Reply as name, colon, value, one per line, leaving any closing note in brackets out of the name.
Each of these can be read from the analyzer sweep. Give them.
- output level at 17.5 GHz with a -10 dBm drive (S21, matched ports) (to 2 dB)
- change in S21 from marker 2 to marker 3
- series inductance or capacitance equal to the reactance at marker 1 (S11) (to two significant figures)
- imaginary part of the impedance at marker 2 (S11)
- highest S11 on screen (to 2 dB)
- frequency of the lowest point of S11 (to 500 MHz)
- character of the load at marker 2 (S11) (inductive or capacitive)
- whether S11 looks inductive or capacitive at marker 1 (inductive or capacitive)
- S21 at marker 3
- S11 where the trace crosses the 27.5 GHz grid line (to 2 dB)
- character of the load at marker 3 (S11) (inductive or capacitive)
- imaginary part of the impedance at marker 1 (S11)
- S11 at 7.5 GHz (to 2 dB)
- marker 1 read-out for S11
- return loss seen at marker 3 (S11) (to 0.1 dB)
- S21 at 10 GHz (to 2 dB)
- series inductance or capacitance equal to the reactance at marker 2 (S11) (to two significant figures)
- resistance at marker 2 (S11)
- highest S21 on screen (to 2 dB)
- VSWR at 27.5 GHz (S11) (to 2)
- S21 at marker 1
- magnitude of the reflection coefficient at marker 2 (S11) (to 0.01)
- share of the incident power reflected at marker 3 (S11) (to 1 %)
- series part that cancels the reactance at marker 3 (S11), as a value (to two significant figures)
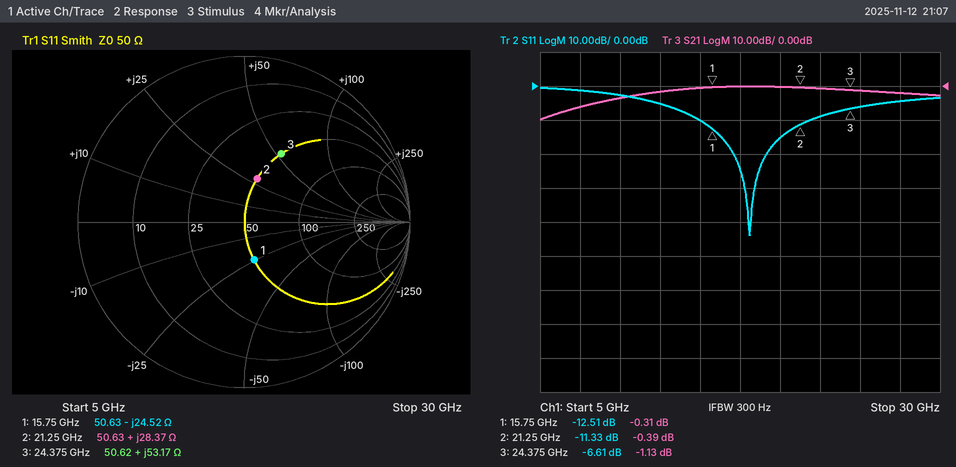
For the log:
output level at 17.5 GHz with a -10 dBm drive (S21, matched ports): -10 dBm
change in S21 from marker 2 to marker 3: -0.74 dB
series inductance or capacitance equal to the reactance at marker 1 (S11): 410 fF
imaginary part of the impedance at marker 2: +28.37 Ω
highest S11 on screen: 0 dB
frequency of the lowest point of S11: 18.0 GHz
character of the load at marker 2 (S11): inductive
whether S11 looks inductive or capacitive at marker 1: capacitive
S21 at marker 3: -1.13 dB
S11 where the trace crosses the 27.5 GHz grid line: -4 dB
character of the load at marker 3 (S11): inductive
imaginary part of the impedance at marker 1: -24.52 Ω
S11 at 7.5 GHz: -2 dB
marker 1 read-out for S11: -12.51 dB
return loss seen at marker 3 (S11): 6.6 dB
S21 at 10 GHz: -4 dB
series inductance or capacitance equal to the reactance at marker 2 (S11): 210 pH
resistance at marker 2: 50.63 Ω
highest S21 on screen: 0 dB
VSWR at 27.5 GHz (S11): 4
S21 at marker 1: -0.31 dB
magnitude of the reflection coefficient at marker 2 (S11): 0.27
share of the incident power reflected at marker 3 (S11): 22 %
series part that cancels the reactance at marker 3 (S11), as a value: 120 fF
